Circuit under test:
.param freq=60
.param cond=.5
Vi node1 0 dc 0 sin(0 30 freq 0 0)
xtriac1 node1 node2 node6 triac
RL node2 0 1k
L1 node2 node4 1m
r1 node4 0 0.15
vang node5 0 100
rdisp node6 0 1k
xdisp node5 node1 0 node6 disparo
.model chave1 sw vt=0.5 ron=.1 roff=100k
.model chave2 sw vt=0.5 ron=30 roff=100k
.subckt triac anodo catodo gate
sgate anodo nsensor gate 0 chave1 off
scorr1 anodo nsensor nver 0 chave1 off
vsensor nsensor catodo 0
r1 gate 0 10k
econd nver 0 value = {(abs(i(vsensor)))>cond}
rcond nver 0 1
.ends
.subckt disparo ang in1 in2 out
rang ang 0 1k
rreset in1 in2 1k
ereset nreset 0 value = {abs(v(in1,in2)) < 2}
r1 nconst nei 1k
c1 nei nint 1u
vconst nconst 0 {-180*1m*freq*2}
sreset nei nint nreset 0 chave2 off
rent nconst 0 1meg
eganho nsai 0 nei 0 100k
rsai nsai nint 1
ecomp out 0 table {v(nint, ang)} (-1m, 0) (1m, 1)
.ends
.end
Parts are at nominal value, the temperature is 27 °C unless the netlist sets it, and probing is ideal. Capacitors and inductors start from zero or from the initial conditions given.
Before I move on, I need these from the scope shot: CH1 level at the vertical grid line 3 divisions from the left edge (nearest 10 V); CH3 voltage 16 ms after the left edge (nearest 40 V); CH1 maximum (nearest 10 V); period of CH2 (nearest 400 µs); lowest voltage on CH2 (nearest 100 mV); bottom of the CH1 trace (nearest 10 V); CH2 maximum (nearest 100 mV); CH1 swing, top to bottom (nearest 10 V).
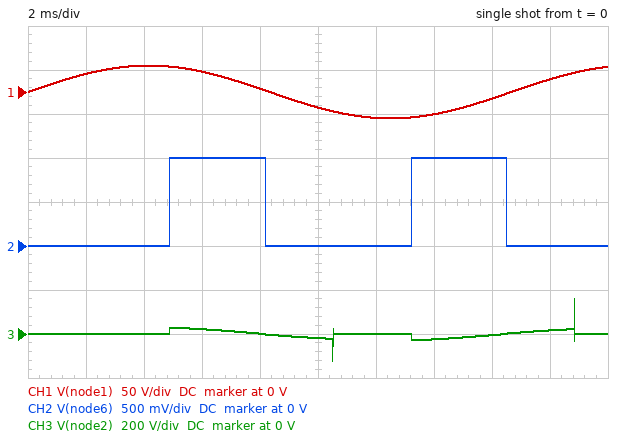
20 V
0 V
30 V
8.4 ms
0 V
-30 V
1.0 V
60 V
